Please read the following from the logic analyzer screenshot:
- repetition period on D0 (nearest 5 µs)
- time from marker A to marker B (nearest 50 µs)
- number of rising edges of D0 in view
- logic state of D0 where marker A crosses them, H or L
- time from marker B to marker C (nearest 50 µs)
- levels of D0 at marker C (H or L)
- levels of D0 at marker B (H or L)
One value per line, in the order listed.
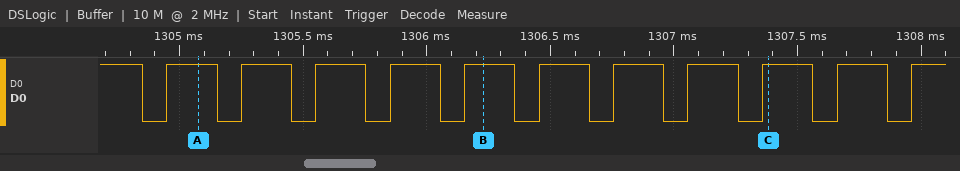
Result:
300 µs
1150 µs
11
D0=H
1150 µs
D0=H
D0=H
